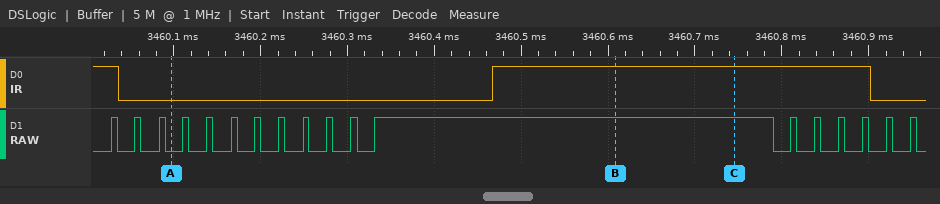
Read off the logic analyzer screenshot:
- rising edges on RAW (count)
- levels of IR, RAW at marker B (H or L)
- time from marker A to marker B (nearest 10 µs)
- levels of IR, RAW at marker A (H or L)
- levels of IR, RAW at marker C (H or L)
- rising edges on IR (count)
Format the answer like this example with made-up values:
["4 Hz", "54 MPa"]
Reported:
["18", "IR=H, RAW=H", "510 µs", "IR=L, RAW=L", "IR=H, RAW=H", "1"]
